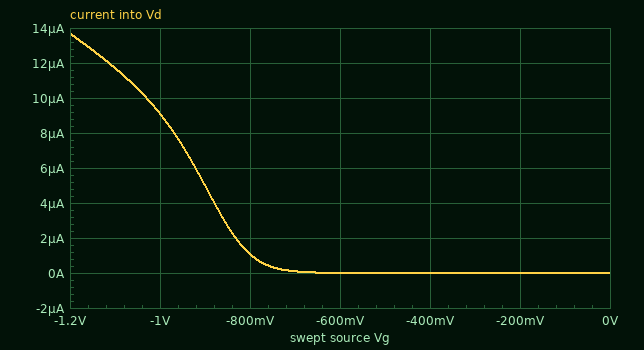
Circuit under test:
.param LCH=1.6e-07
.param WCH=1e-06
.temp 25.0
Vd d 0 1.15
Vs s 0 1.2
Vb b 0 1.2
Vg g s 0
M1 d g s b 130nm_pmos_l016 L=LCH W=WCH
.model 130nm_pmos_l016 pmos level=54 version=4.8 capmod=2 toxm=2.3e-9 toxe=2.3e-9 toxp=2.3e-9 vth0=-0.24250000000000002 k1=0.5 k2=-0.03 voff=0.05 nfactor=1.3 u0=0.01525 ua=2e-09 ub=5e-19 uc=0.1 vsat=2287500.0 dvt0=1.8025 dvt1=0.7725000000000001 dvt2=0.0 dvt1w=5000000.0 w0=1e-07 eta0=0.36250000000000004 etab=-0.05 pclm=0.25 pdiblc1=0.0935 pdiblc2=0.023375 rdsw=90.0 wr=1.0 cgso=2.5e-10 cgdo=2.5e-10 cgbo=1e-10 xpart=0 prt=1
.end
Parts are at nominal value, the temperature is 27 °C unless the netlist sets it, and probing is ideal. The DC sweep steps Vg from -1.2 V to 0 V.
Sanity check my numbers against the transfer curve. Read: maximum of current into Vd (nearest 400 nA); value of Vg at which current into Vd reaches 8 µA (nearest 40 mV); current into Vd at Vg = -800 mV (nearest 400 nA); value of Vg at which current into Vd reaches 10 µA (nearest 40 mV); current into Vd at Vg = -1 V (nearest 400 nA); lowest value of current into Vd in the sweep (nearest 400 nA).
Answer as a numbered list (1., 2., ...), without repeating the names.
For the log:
1. 13.6 µA
2. -960 mV
3. 1.2 µA
4. -1.04 V
5. 9.2 µA
6. 0 A
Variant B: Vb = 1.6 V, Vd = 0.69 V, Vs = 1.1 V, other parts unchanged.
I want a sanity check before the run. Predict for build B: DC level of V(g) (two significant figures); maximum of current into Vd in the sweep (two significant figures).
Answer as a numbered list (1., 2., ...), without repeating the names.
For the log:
1. 1.1 V
2. 1.3 mA
